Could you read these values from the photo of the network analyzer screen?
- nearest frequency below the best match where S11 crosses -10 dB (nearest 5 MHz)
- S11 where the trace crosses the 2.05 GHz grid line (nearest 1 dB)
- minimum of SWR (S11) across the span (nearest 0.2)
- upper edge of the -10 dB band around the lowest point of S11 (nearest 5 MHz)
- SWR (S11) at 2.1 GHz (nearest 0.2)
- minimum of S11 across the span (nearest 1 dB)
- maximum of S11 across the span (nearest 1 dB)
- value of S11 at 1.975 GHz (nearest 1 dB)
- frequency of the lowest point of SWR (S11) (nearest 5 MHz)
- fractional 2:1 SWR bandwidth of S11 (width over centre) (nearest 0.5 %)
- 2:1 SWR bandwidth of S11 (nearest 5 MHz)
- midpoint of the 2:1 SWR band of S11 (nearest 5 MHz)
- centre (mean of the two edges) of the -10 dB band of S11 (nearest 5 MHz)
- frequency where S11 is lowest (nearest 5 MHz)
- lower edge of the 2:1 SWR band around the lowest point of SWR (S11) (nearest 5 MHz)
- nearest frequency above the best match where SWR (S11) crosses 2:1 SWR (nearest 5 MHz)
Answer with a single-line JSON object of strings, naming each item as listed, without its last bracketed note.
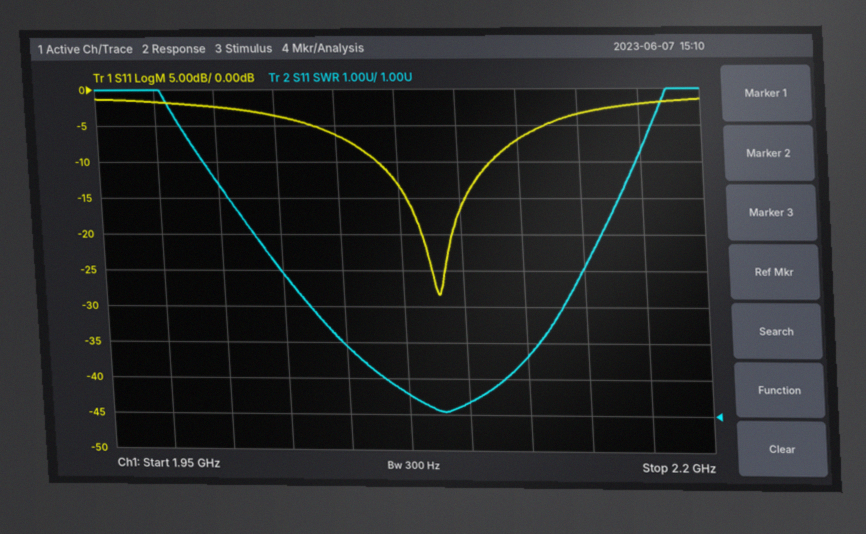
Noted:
{"nearest frequency below the best match where S11 crosses -10 dB": "2.065 GHz", "S11 where the trace crosses the 2.05 GHz grid line": "-6 dB", "minimum of SWR (S11) across the span": "1.0", "upper edge of the -10 dB band around the lowest point of S11": "2.115 GHz", "SWR (S11) at 2.1 GHz": "1.4", "minimum of S11 across the span": "-28 dB", "maximum of S11 across the span": "-1 dB", "value of S11 at 1.975 GHz": "-2 dB", "frequency of the lowest point of SWR (S11)": "2.090 GHz", "fractional 2:1 SWR bandwidth of S11 (width over centre)": "2.5 %", "2:1 SWR bandwidth of S11": "50 MHz", "midpoint of the 2:1 SWR band of S11": "2.090 GHz", "centre (mean of the two edges) of the -10 dB band of S11": "2.090 GHz", "frequency where S11 is lowest": "2.090 GHz", "lower edge of the 2:1 SWR band around the lowest point of SWR (S11)": "2.065 GHz", "nearest frequency above the best match where SWR (S11) crosses 2:1 SWR": "2.115 GHz"}
